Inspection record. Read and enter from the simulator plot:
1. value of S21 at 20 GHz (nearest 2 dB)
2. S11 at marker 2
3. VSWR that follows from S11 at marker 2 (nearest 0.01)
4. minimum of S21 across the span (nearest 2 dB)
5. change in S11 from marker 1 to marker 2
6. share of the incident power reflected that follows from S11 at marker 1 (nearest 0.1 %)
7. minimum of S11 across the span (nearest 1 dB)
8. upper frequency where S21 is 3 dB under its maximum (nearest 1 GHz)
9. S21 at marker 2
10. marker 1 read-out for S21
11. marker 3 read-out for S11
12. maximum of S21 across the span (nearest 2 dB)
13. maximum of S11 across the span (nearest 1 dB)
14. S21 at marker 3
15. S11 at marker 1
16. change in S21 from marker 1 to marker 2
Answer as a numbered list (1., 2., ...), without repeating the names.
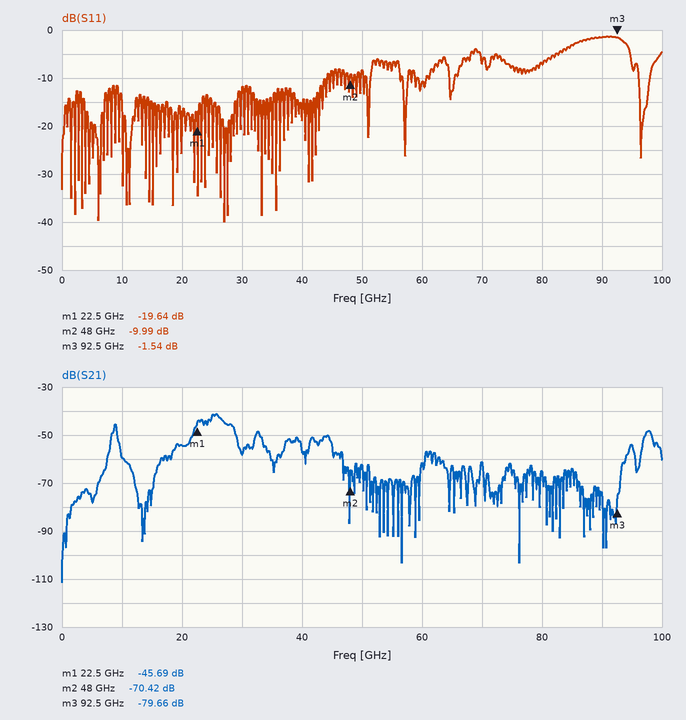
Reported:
1. -54 dB
2. -9.99 dB
3. 1.93
4. -112 dB
5. 9.65 dB
6. 1.1 %
7. -40 dB
8. 27 GHz
9. -70.42 dB
10. -45.69 dB
11. -1.54 dB
12. -42 dB
13. -1 dB
14. -79.66 dB
15. -19.64 dB
16. -24.73 dB
